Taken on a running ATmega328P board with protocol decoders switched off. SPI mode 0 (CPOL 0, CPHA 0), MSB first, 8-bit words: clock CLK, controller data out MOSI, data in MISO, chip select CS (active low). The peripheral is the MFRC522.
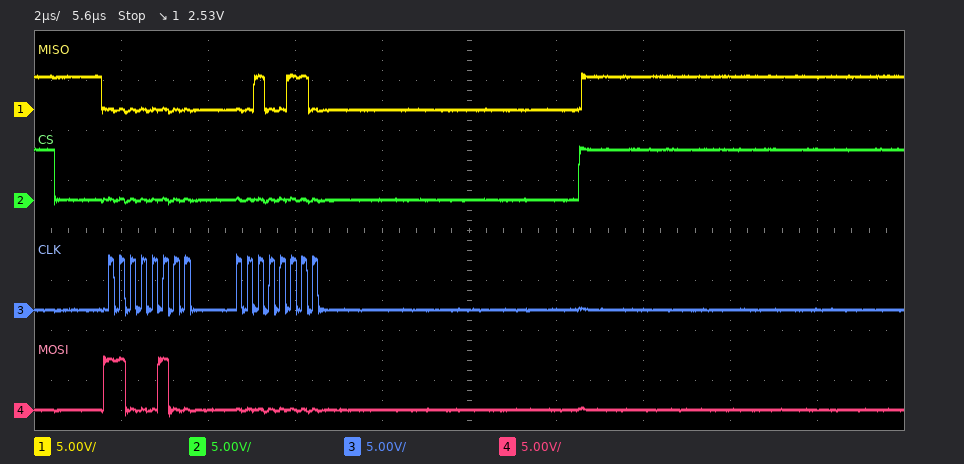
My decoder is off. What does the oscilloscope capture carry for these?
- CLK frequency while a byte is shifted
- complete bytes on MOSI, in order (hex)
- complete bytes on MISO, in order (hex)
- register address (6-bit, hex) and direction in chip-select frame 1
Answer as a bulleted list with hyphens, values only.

- 4 MHz
- C4 00
- 00 26
- 0x22 read
